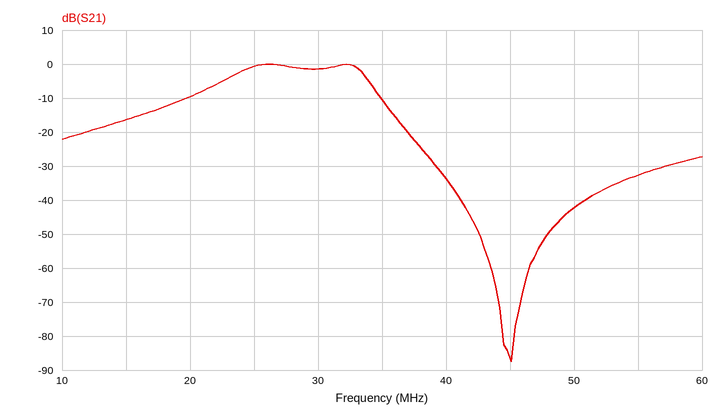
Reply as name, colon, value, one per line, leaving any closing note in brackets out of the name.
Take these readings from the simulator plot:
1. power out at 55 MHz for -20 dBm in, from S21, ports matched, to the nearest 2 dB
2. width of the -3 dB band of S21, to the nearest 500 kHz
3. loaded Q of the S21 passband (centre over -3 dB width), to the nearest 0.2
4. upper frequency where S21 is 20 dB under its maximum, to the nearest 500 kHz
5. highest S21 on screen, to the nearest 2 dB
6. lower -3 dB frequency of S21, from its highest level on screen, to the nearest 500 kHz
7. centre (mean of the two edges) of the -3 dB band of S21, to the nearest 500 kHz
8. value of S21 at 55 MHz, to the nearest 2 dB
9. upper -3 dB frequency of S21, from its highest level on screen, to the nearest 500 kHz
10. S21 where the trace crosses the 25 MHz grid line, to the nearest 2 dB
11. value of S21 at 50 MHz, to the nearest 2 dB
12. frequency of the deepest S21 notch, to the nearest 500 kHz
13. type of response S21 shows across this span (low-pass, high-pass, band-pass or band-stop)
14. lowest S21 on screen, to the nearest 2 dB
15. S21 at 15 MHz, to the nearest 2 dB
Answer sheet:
power out at 55 MHz for -20 dBm in, from S21, ports matched, to the nearest 2 dB: -52 dBm
width of the -3 dB band of S21, to the nearest 500 kHz: 10.0 MHz
loaded Q of the S21 passband (centre over -3 dB width), to the nearest 0.2: 2.8
upper frequency where S21 is 20 dB under its maximum, to the nearest 500 kHz: 37.0 MHz
highest S21 on screen, to the nearest 2 dB: 0 dB
lower -3 dB frequency of S21, from its highest level on screen, to the nearest 500 kHz: 23.5 MHz
centre (mean of the two edges) of the -3 dB band of S21, to the nearest 500 kHz: 28.5 MHz
value of S21 at 55 MHz, to the nearest 2 dB: -32 dB
upper -3 dB frequency of S21, from its highest level on screen, to the nearest 500 kHz: 33.5 MHz
S21 where the trace crosses the 25 MHz grid line, to the nearest 2 dB: 0 dB
value of S21 at 50 MHz, to the nearest 2 dB: -42 dB
frequency of the deepest S21 notch, to the nearest 500 kHz: 45.0 MHz
type of response S21 shows across this span: band-pass
lowest S21 on screen, to the nearest 2 dB: -88 dB
S21 at 15 MHz, to the nearest 2 dB: -16 dB
